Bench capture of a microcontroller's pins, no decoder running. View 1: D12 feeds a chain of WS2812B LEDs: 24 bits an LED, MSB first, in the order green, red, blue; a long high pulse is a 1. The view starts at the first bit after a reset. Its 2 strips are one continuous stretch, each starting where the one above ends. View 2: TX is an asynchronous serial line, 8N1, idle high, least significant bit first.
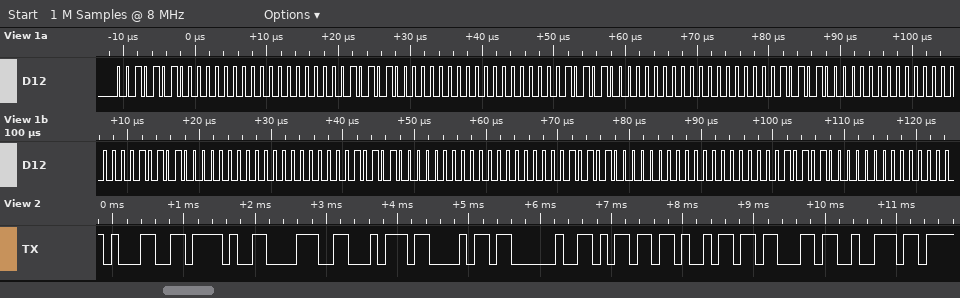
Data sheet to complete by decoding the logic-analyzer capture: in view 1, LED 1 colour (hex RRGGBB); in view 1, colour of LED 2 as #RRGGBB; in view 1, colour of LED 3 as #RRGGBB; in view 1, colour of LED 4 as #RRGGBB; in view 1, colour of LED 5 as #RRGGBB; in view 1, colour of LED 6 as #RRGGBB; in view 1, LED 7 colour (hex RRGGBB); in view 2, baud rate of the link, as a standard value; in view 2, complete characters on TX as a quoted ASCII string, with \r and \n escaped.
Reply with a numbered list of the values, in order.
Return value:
1. #002A00
2. #002A00
3. #002A00
4. #002A00
5. #002A00
6. #002A00
7. #002A00
8. 9600 baud
9. "1/8th micr"
